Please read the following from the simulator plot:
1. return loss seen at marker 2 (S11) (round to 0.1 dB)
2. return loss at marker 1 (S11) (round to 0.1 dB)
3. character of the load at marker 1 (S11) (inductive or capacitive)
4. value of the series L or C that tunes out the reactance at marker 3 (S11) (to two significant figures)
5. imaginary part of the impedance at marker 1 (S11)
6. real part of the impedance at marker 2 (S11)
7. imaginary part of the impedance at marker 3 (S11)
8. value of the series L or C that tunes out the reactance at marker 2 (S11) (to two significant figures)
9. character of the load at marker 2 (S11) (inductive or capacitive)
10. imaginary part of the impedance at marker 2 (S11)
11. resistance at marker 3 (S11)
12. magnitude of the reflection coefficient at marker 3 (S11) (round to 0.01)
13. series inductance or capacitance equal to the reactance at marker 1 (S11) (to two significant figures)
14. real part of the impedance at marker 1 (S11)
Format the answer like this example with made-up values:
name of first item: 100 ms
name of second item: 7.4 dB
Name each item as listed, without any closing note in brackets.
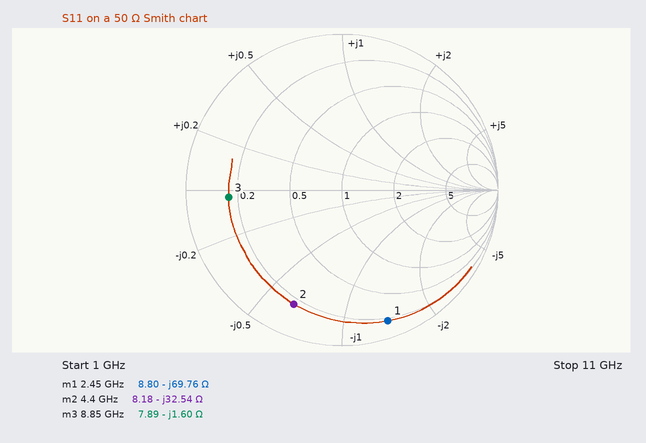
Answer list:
return loss seen at marker 2 (S11): 2.0 dB
return loss at marker 1 (S11): 1.0 dB
character of the load at marker 1 (S11): capacitive
value of the series L or C that tunes out the reactance at marker 3 (S11): 29 pH
imaginary part of the impedance at marker 1: -69.76 Ω
real part of the impedance at marker 2: 8.18 Ω
imaginary part of the impedance at marker 3: -1.60 Ω
value of the series L or C that tunes out the reactance at marker 2 (S11): 1.2 nH
character of the load at marker 2 (S11): capacitive
imaginary part of the impedance at marker 2: -32.54 Ω
resistance at marker 3: 7.89 Ω
magnitude of the reflection coefficient at marker 3 (S11): 0.73
series inductance or capacitance equal to the reactance at marker 1 (S11): 930 fF
real part of the impedance at marker 1: 8.80 Ω
